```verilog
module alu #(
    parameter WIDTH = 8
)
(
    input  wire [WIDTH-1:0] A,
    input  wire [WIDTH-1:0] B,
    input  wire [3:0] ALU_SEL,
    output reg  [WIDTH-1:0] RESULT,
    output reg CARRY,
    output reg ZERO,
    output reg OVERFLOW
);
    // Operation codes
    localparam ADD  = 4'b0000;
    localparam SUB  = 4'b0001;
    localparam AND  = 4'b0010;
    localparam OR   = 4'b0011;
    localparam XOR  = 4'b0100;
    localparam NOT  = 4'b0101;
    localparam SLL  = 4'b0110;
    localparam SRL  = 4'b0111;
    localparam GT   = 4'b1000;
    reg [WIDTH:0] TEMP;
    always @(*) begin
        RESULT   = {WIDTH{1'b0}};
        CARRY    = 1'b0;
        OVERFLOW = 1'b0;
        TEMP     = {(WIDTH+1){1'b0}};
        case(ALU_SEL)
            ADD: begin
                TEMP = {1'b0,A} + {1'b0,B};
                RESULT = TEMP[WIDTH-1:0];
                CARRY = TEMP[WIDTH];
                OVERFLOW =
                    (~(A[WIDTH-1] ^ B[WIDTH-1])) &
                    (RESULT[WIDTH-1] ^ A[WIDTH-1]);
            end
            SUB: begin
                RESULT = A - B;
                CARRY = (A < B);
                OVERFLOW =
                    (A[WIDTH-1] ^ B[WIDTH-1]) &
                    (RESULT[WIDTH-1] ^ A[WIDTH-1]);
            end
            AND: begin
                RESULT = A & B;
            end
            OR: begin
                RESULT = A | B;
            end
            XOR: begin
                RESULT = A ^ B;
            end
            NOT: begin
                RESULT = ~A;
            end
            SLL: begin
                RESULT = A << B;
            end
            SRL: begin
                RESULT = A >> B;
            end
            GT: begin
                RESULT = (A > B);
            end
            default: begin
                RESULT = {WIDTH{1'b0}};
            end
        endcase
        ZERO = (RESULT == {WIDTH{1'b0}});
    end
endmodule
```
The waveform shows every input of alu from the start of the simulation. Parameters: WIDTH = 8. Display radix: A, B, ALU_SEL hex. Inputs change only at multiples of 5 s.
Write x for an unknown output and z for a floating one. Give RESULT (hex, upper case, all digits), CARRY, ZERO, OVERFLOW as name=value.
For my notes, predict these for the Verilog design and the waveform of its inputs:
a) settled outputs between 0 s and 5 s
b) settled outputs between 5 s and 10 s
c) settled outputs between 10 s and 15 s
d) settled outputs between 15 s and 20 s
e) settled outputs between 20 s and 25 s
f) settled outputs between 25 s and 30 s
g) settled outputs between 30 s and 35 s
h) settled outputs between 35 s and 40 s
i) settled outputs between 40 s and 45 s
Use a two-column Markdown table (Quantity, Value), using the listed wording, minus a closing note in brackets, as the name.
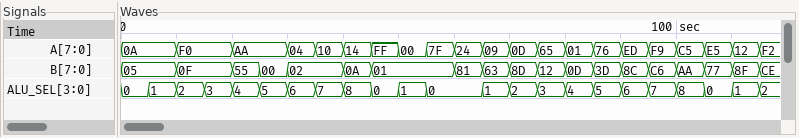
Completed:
| Quantity | Value |
|---|---|
| settled outputs between 0 s and 5 s | RESULT=0F, CARRY=0, ZERO=0, OVERFLOW=0 |
| settled outputs between 5 s and 10 s | RESULT=05, CARRY=0, ZERO=0, OVERFLOW=0 |
| settled outputs between 10 s and 15 s | RESULT=00, CARRY=0, ZERO=1, OVERFLOW=0 |
| settled outputs between 15 s and 20 s | RESULT=FF, CARRY=0, ZERO=0, OVERFLOW=0 |
| settled outputs between 20 s and 25 s | RESULT=FF, CARRY=0, ZERO=0, OVERFLOW=0 |
| settled outputs between 25 s and 30 s | RESULT=55, CARRY=0, ZERO=0, OVERFLOW=0 |
| settled outputs between 30 s and 35 s | RESULT=10, CARRY=0, ZERO=0, OVERFLOW=0 |
| settled outputs between 35 s and 40 s | RESULT=04, CARRY=0, ZERO=0, OVERFLOW=0 |
| settled outputs between 40 s and 45 s | RESULT=01, CARRY=0, ZERO=0, OVERFLOW=0 |
